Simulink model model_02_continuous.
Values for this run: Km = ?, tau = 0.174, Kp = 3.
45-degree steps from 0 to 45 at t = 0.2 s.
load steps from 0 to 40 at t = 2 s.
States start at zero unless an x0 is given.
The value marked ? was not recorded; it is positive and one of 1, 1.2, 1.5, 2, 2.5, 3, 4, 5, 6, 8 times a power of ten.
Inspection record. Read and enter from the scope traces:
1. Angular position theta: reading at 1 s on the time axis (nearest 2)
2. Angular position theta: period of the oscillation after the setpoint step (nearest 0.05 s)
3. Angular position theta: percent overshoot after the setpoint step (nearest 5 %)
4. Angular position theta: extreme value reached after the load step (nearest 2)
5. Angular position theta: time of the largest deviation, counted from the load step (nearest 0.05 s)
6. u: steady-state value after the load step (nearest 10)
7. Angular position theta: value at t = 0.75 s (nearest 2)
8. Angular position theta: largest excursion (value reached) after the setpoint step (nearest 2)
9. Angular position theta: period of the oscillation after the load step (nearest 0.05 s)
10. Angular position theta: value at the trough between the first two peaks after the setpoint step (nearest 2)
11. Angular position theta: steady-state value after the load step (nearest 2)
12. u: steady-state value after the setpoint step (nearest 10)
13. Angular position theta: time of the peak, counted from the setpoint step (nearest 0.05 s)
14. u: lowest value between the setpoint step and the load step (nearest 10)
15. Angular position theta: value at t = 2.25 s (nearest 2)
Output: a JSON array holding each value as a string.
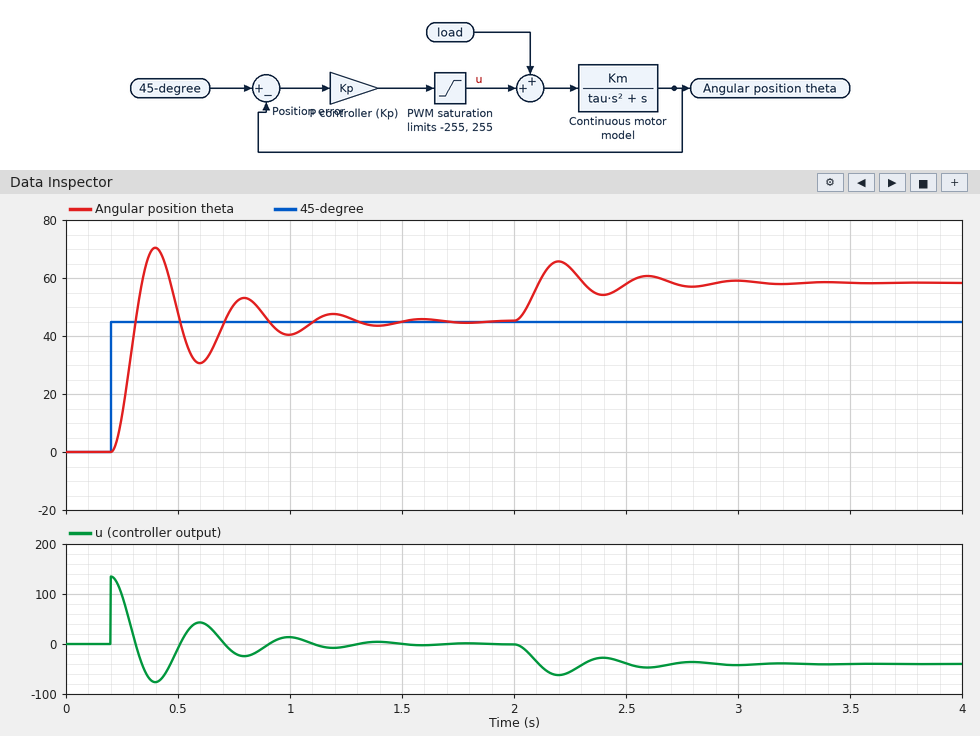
["40", "0.40 s", "55 %", "66", "0.20 s", "-40", "50", "70", "0.40 s", "30", "58", "0", "0.20 s", "-80", "64"]
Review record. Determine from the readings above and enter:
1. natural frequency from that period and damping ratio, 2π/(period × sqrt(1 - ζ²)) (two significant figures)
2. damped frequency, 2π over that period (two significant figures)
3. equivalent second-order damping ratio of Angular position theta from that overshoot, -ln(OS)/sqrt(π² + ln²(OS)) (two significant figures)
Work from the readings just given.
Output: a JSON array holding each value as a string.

["16 rad/s", "16 rad/s", "0.19"]
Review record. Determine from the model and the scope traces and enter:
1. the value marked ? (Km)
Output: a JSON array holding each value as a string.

["15"]
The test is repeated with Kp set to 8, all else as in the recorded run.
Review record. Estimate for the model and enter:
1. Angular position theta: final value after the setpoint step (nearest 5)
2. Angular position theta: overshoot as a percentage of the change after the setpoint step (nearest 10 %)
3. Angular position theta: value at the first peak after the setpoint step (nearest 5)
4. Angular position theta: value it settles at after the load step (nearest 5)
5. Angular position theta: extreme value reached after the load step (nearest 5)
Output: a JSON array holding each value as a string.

["45", "70 %", "75", "50", "55"]
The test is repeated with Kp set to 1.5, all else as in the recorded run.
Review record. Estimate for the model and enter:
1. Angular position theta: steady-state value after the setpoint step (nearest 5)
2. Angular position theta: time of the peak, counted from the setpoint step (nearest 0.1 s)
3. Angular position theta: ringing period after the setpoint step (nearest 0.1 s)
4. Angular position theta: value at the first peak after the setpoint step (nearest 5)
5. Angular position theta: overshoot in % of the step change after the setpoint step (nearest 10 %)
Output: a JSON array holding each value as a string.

["45", "0.3 s", "0.6 s", "65", "40 %"]
